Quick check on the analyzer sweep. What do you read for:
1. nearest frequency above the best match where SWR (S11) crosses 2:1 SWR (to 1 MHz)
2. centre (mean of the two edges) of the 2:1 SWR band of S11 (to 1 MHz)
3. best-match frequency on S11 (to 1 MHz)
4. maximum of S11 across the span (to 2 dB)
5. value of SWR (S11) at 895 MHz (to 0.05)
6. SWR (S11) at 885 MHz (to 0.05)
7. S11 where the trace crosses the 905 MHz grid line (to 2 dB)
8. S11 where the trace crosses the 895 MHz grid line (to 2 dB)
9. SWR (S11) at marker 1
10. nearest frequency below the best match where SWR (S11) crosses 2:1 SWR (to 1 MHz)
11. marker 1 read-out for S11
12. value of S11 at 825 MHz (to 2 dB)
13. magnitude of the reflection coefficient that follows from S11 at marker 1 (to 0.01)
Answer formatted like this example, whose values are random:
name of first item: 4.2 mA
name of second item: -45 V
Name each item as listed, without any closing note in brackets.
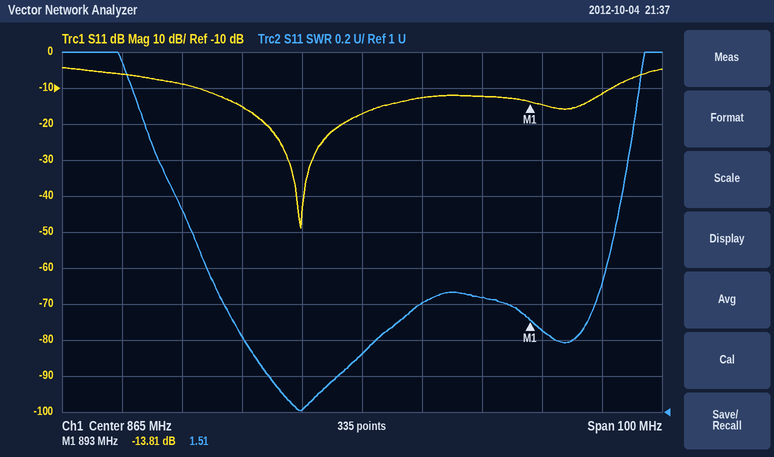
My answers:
nearest frequency above the best match where SWR (S11) crosses 2:1 SWR: 907 MHz
centre (mean of the two edges) of the 2:1 SWR band of S11: 872 MHz
best-match frequency on S11: 855 MHz
maximum of S11 across the span: -4 dB
value of SWR (S11) at 895 MHz: 1.45
SWR (S11) at 885 MHz: 1.65
S11 where the trace crosses the 905 MHz grid line: -12 dB
S11 where the trace crosses the 895 MHz grid line: -14 dB
SWR (S11) at marker 1: 1.51
nearest frequency below the best match where SWR (S11) crosses 2:1 SWR: 837 MHz
marker 1 read-out for S11: -13.81 dB
value of S11 at 825 MHz: -6 dB
magnitude of the reflection coefficient that follows from S11 at marker 1: 0.20
